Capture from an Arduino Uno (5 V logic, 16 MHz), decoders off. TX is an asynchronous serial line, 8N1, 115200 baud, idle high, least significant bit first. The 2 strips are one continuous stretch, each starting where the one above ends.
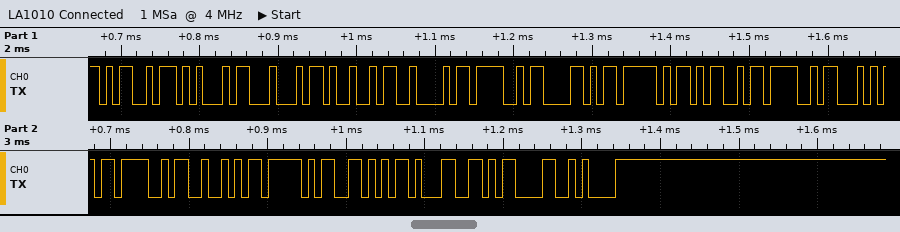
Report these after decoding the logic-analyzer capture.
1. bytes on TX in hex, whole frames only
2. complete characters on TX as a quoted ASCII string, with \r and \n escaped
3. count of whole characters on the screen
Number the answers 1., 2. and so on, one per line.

1. 4D 45 44 49 42 4F 58 5F 4D 4F 54 4F 52 5F 56 31 0D 0A
2. "MEDIBOX_MOTOR_V1\r\n"
3. 18
